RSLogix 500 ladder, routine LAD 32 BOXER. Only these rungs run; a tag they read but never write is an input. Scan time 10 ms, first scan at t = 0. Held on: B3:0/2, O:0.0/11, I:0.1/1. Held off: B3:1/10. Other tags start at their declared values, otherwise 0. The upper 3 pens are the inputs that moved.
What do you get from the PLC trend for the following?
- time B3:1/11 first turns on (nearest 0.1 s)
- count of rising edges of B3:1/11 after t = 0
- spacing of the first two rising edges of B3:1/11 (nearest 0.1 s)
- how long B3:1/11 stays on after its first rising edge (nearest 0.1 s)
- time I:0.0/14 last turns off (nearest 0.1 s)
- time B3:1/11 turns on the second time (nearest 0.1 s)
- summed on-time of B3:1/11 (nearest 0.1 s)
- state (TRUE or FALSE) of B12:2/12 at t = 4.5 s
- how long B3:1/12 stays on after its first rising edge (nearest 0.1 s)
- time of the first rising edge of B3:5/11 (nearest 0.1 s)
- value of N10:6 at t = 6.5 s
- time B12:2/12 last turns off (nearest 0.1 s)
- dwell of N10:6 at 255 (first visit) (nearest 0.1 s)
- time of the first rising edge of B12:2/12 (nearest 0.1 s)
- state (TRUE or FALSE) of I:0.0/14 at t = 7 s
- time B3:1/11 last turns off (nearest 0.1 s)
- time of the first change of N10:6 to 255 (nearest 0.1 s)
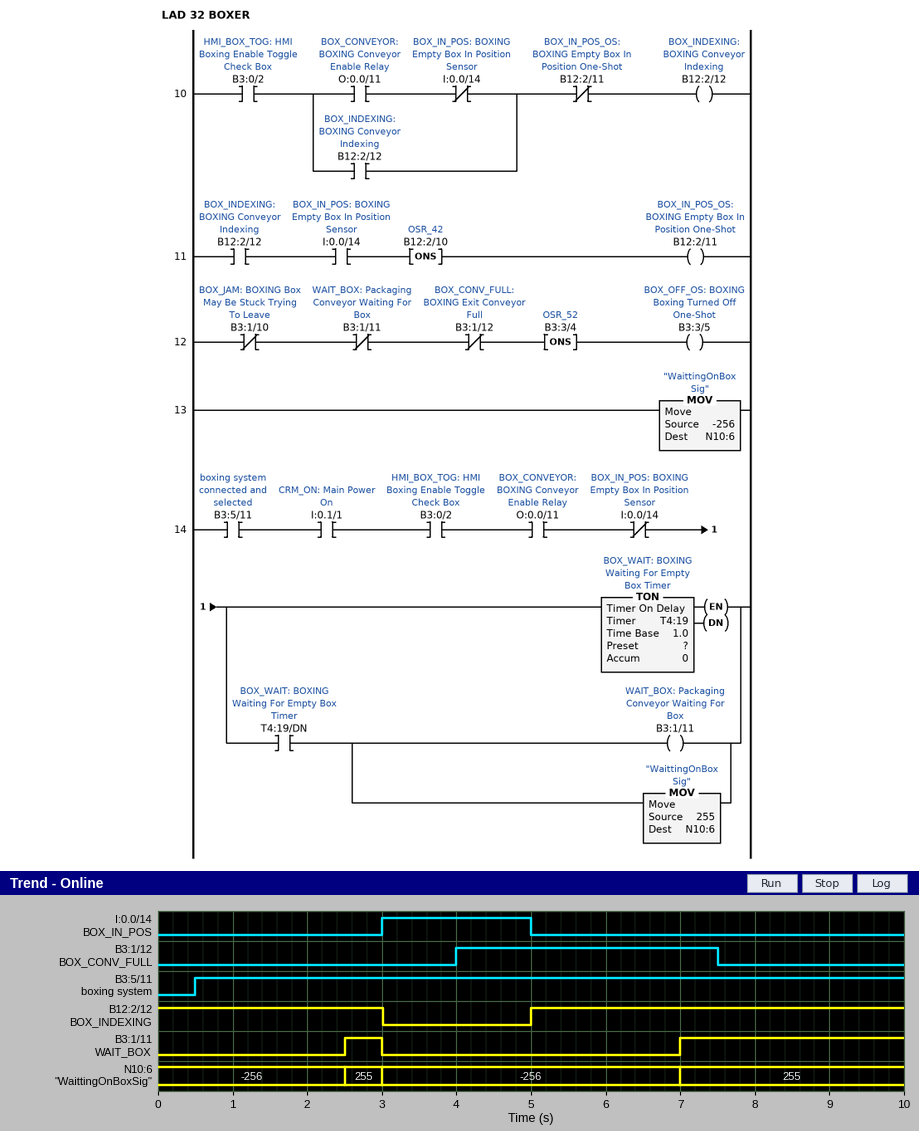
2.5 s
2
4.5 s
0.5 s
5.0 s
7.0 s
3.5 s
FALSE
3.5 s
0.5 s
-256
3.0 s
0.5 s
5.0 s
FALSE
3.0 s
2.5 s
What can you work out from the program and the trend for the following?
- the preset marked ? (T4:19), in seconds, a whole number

2 s
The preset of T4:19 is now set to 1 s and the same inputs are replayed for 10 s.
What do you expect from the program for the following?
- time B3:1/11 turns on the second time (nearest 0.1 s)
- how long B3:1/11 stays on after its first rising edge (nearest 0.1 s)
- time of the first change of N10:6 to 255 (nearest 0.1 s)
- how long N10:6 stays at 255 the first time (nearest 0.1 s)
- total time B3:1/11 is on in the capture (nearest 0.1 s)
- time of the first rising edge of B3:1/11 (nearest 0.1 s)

6.0 s
1.5 s
1.5 s
1.5 s
5.5 s
1.5 s
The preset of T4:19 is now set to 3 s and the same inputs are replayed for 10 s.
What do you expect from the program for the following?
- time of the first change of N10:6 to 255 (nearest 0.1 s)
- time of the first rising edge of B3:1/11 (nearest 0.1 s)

8.0 s
8.0 s
